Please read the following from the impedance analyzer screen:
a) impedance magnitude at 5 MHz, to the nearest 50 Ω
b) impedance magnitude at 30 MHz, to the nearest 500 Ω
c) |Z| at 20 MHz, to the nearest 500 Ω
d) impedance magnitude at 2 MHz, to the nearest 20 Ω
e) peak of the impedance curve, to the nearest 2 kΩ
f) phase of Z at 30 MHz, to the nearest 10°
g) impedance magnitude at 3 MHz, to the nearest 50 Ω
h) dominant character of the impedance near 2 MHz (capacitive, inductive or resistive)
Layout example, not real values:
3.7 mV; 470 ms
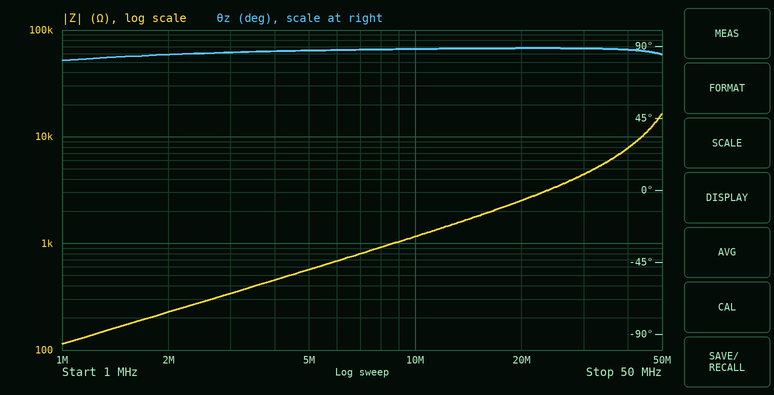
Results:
550 Ω; 4.5 kΩ; 2.5 kΩ; 220 Ω; 16 kΩ; 90°; 350 Ω; inductive
